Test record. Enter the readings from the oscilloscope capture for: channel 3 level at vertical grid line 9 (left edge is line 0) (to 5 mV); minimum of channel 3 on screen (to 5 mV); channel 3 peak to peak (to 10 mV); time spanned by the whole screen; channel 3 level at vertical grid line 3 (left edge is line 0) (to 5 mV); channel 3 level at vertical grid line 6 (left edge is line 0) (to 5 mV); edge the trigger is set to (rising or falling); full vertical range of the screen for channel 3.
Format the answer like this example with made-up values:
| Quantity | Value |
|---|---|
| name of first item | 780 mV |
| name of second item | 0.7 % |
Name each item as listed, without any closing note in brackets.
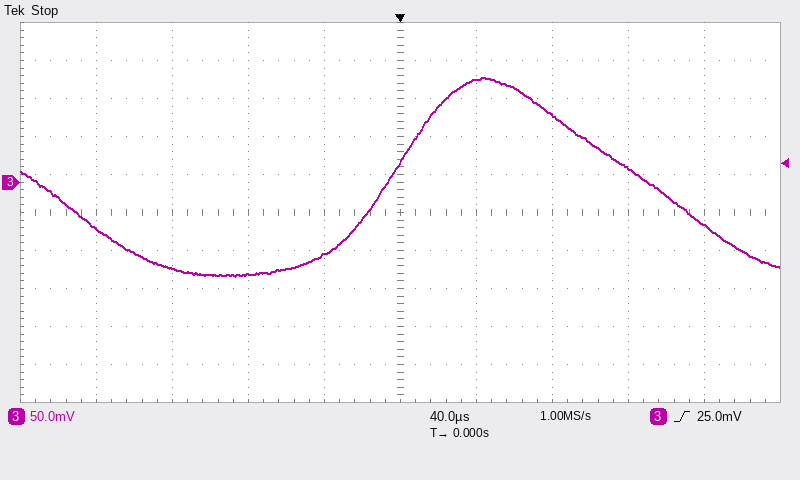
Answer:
| Quantity | Value |
|---|---|
| channel 3 level at vertical grid line 9 (left edge is line 0) | -55 mV |
| minimum of channel 3 on screen | -125 mV |
| channel 3 peak to peak | 260 mV |
| time spanned by the whole screen | 400 µs |
| channel 3 level at vertical grid line 3 (left edge is line 0) | -120 mV |
| channel 3 level at vertical grid line 6 (left edge is line 0) | 135 mV |
| edge the trigger is set to | rising |
| full vertical range of the screen for channel 3 | 500 mV |
